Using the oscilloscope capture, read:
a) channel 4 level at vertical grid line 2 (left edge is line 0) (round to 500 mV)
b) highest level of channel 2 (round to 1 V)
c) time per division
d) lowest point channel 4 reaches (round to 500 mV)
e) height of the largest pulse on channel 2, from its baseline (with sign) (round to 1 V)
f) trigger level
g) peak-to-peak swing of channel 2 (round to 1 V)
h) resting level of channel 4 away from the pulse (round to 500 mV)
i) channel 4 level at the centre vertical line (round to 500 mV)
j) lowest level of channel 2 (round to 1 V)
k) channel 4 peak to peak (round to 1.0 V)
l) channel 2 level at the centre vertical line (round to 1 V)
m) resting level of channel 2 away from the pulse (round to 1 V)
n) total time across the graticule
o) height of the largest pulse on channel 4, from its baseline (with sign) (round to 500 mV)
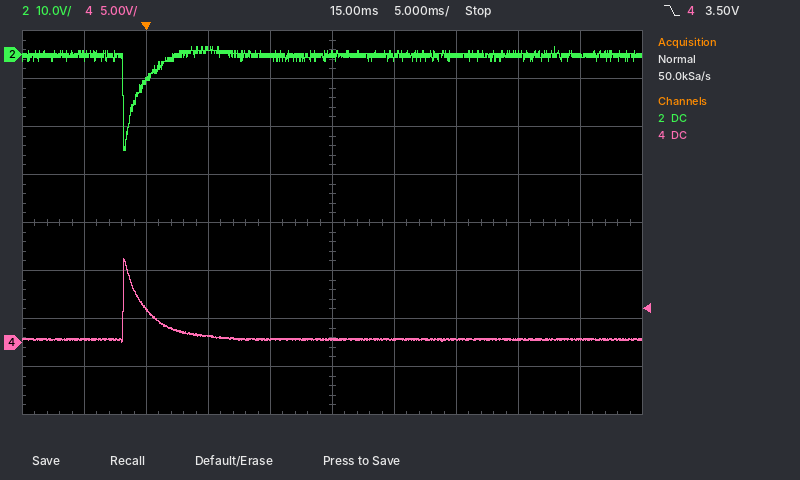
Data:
3.5 V
2 V
5 ms
0.0 V
-20 V
3.50 V
22 V
500 mV
500 mV
-20 V
9.0 V
0 V
0 V
50 ms
+8.5 V
